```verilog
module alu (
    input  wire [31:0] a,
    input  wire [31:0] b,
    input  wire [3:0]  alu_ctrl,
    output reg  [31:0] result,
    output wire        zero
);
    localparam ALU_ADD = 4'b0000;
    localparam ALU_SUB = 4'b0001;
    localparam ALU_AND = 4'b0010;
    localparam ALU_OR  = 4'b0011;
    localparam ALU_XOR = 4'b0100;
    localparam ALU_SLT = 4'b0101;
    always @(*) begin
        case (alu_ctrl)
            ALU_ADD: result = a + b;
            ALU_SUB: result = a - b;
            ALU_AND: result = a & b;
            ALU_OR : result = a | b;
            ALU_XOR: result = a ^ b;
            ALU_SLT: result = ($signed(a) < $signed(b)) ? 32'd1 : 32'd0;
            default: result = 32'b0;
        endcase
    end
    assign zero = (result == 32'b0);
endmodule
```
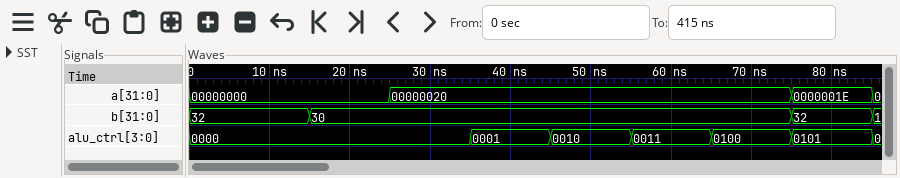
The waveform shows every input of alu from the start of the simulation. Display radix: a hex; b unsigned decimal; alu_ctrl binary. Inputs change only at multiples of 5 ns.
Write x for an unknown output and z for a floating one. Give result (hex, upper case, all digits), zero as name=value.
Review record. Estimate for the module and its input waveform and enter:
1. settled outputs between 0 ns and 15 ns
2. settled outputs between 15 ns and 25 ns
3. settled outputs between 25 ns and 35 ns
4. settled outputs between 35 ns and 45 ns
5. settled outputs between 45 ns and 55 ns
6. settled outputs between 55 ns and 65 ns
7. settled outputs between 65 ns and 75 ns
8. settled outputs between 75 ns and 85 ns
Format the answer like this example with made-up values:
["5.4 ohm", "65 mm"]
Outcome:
["result=00000020, zero=0", "result=0000001E, zero=0", "result=0000003E, zero=0", "result=00000002, zero=0", "result=00000000, zero=1", "result=0000003E, zero=0", "result=0000003E, zero=0", "result=00000001, zero=0"]
